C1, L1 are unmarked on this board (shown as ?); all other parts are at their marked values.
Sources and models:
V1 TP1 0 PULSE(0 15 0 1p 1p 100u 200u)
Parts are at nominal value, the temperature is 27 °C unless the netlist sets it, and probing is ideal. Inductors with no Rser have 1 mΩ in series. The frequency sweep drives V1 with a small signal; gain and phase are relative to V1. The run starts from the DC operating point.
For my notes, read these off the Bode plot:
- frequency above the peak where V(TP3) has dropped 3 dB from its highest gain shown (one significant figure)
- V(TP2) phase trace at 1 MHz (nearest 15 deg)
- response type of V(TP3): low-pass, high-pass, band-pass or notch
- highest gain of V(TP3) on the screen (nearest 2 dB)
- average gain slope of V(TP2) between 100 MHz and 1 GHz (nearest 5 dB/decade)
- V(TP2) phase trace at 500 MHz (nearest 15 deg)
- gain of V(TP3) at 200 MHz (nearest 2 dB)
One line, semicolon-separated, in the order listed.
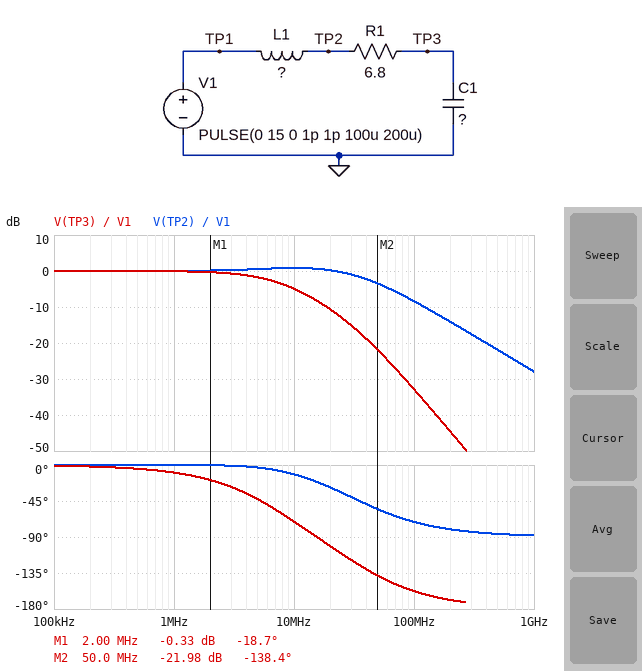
7 MHz; 0 deg; low-pass; 0 dB; -20 dB/decade; -90 deg; -44 dB
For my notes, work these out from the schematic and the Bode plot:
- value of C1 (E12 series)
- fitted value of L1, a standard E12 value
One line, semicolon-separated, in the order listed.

3.9 nF; 27 nH
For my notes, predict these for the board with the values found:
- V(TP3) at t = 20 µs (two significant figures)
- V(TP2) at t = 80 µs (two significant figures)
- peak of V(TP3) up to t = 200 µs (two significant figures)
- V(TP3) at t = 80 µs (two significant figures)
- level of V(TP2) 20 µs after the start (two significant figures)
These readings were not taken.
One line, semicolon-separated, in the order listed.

15 V; 15 V; 15 V; 15 V; 15 V
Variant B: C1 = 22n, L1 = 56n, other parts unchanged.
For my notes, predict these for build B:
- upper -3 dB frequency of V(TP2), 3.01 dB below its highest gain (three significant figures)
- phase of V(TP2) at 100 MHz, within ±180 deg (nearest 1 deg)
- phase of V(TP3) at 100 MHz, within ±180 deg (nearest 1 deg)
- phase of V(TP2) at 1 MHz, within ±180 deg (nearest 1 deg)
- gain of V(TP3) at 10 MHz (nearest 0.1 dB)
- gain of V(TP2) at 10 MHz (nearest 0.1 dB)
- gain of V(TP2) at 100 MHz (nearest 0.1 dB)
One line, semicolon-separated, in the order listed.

18.9 MHz; -80 deg; -169 deg; -1 deg; -20.1 dB; -0.6 dB; -14.4 dB
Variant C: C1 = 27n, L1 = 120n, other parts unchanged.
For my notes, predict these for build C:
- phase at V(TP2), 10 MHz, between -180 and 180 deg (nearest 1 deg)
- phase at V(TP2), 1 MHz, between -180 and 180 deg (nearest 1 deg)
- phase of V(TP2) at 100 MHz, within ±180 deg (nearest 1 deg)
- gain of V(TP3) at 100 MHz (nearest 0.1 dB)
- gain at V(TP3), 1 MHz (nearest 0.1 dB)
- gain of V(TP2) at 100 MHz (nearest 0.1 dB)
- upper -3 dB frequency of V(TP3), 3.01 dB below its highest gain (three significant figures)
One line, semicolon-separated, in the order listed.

-51 deg; -4 deg; -85 deg; -62.2 dB; -3.2 dB; -20.9 dB; 958 kHz
